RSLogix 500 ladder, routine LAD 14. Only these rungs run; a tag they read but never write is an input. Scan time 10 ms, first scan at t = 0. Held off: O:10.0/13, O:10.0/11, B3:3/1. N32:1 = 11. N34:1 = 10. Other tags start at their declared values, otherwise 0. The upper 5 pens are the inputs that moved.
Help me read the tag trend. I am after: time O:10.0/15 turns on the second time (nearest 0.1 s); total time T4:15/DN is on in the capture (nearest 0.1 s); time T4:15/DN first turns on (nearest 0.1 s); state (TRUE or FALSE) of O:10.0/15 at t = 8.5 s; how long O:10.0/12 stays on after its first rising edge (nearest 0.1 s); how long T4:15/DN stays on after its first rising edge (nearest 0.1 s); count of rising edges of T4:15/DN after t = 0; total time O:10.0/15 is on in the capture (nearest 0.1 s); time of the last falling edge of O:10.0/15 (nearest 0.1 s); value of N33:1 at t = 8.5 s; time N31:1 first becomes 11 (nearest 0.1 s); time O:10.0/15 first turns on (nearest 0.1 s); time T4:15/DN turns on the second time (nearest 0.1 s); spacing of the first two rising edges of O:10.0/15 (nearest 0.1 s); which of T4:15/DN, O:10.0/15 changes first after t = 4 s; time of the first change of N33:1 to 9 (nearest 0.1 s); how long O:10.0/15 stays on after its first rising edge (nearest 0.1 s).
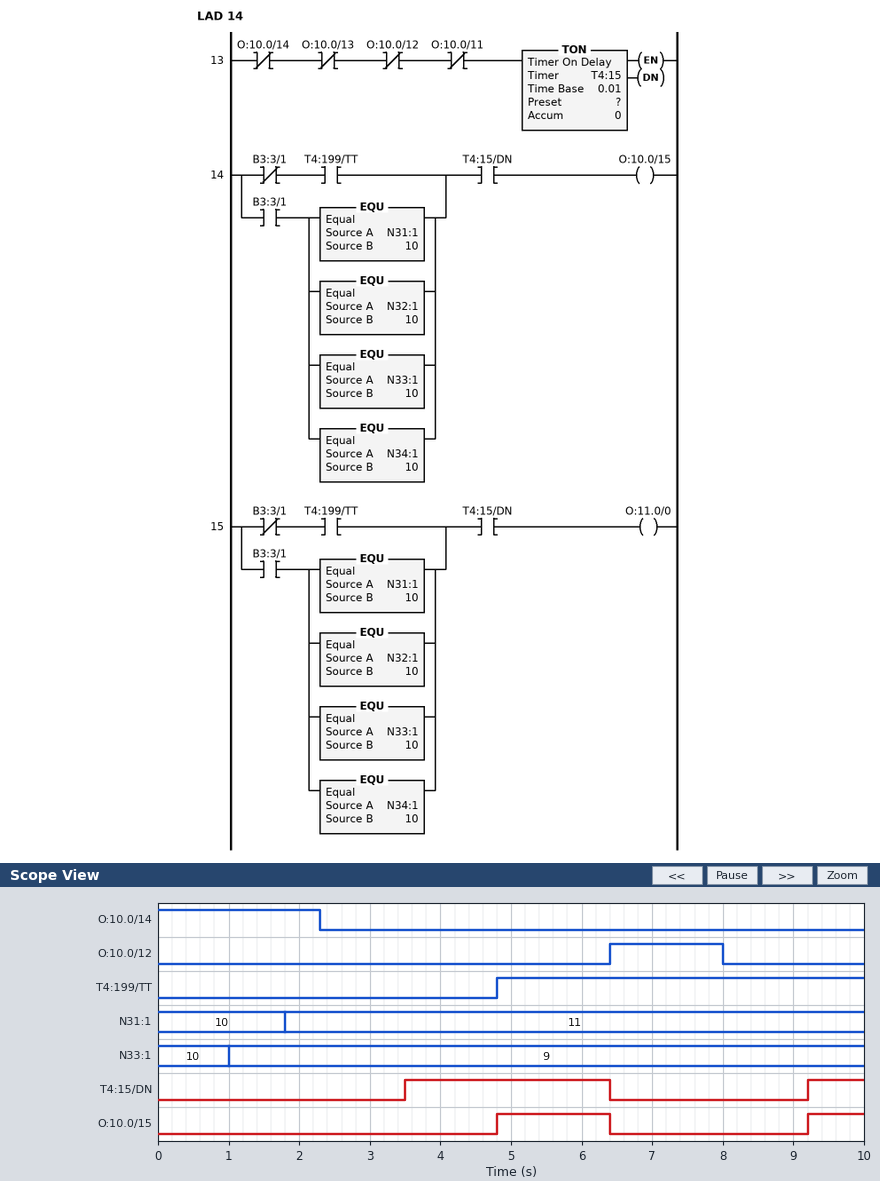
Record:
9.2 s
3.7 s
3.5 s
FALSE
1.6 s
2.9 s
2
2.4 s
6.4 s
9
1.8 s
4.8 s
9.2 s
4.4 s
O:10.0/15
1.0 s
1.6 s
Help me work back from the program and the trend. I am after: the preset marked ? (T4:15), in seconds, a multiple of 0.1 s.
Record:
1.2 s
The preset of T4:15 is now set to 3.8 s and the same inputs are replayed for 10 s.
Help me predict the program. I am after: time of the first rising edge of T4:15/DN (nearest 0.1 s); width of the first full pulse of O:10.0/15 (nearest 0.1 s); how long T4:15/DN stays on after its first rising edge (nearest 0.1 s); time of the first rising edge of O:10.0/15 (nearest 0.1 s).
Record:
6.1 s
0.3 s
0.3 s
6.1 s
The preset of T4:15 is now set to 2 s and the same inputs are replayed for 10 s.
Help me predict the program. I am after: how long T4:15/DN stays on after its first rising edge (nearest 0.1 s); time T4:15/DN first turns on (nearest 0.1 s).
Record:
2.1 s
4.3 s
